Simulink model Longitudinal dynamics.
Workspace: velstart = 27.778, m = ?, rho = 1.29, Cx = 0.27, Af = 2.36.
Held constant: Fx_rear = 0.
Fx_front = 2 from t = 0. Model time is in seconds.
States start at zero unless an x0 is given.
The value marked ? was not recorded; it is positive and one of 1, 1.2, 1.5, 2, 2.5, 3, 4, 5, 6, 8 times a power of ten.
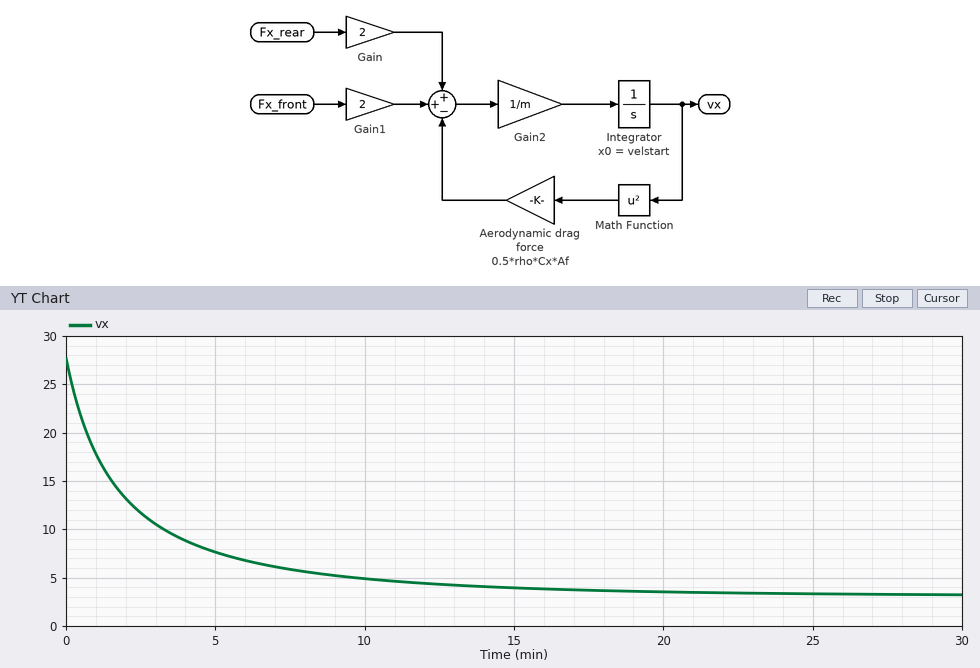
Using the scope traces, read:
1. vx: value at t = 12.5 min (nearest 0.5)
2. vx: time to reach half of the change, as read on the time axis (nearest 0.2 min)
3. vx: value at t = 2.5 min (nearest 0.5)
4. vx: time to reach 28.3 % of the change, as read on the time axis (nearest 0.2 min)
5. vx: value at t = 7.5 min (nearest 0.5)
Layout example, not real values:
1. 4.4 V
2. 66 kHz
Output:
1. 4.5
2. 1.4 min
3. 11.5
4. 0.6 min
5. 6.0
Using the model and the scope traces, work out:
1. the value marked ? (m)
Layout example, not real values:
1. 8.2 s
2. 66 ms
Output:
1. 1200
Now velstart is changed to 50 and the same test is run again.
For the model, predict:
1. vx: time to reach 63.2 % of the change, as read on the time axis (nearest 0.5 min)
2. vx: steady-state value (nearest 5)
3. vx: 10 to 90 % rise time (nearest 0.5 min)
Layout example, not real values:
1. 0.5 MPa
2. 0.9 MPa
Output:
1. 1.5 min
2. 5
3. 5.5 min
